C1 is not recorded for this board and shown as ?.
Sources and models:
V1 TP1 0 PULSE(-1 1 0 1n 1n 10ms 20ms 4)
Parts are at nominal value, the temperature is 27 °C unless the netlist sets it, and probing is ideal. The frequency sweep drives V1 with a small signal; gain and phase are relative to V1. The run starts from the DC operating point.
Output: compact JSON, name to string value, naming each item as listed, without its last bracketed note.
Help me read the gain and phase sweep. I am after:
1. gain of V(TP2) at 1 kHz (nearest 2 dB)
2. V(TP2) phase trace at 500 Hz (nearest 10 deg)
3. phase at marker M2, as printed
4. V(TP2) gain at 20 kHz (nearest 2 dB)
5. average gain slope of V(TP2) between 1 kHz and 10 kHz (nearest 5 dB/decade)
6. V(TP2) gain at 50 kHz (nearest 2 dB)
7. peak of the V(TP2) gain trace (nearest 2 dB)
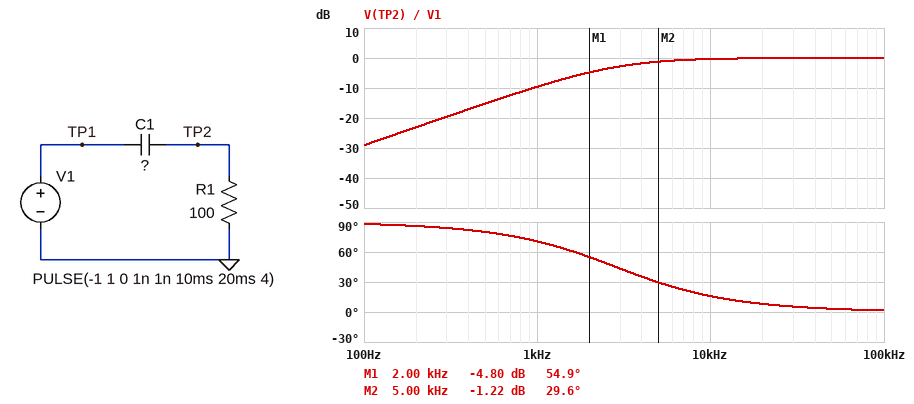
{"gain of V(TP2) at 1 kHz": "-10 dB", "V(TP2) phase trace at 500 Hz": "80 deg", "phase at marker M2, as printed": "29.6 deg", "V(TP2) gain at 20 kHz": "0 dB", "average gain slope of V(TP2) between 1 kHz and 10 kHz": "10 dB/decade", "V(TP2) gain at 50 kHz": "0 dB", "peak of the V(TP2) gain trace": "0 dB"}
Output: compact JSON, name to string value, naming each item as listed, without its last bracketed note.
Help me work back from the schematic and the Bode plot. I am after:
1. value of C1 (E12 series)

{"value of C1": "560 nF"}
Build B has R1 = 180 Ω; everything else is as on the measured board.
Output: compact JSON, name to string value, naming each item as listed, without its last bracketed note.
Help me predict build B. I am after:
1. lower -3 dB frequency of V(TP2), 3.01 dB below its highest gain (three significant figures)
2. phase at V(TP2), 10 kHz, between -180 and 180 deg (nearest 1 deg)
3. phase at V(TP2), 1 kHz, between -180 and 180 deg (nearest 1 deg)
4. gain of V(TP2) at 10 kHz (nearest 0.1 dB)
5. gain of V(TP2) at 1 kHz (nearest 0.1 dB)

{"lower -3 dB frequency of V(TP2), 3.01 dB below its highest gain": "1.58 kHz", "phase at V(TP2), 10 kHz, between -180 and 180 deg": "9 deg", "phase at V(TP2), 1 kHz, between -180 and 180 deg": "58 deg", "gain of V(TP2) at 10 kHz": "-0.1 dB", "gain of V(TP2) at 1 kHz": "-5.4 dB"}
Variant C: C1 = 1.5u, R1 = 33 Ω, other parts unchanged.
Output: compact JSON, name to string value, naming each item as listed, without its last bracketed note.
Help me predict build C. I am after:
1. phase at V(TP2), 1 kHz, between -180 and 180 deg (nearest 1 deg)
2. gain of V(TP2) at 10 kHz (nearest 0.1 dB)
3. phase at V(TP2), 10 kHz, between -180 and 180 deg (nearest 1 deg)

{"phase at V(TP2), 1 kHz, between -180 and 180 deg": "73 deg", "gain of V(TP2) at 10 kHz": "-0.4 dB", "phase at V(TP2), 10 kHz, between -180 and 180 deg": "18 deg"}
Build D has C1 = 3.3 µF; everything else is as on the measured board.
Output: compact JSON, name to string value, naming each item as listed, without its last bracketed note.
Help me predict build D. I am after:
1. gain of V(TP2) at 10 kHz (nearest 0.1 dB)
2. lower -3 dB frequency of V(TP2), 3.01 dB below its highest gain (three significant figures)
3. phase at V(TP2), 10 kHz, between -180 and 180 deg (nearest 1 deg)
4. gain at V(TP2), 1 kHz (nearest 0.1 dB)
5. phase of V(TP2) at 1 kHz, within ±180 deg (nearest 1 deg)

{"gain of V(TP2) at 10 kHz": "0 dB", "lower -3 dB frequency of V(TP2), 3.01 dB below its highest gain": "482 Hz", "phase at V(TP2), 10 kHz, between -180 and 180 deg": "3 deg", "gain at V(TP2), 1 kHz": "-0.9 dB", "phase of V(TP2) at 1 kHz, within ±180 deg": "26 deg"}
